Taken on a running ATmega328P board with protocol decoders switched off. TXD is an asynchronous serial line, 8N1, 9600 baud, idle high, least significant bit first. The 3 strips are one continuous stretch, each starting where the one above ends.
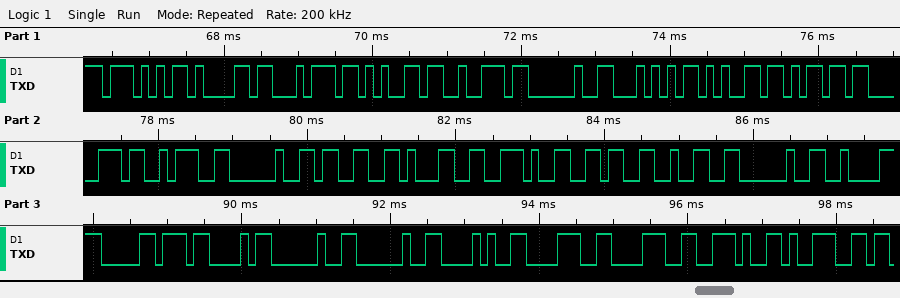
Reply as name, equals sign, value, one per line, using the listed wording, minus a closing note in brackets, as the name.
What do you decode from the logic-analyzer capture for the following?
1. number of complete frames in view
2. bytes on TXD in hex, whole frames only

number of complete frames in view = 28
bytes on TXD in hex, whole frames only = 57 61 74 65 72 20 54 65 6D 70 3A 20 33 31 2E 36 32 20 C2 B0 43 20 20 28 38 38 2E 39
